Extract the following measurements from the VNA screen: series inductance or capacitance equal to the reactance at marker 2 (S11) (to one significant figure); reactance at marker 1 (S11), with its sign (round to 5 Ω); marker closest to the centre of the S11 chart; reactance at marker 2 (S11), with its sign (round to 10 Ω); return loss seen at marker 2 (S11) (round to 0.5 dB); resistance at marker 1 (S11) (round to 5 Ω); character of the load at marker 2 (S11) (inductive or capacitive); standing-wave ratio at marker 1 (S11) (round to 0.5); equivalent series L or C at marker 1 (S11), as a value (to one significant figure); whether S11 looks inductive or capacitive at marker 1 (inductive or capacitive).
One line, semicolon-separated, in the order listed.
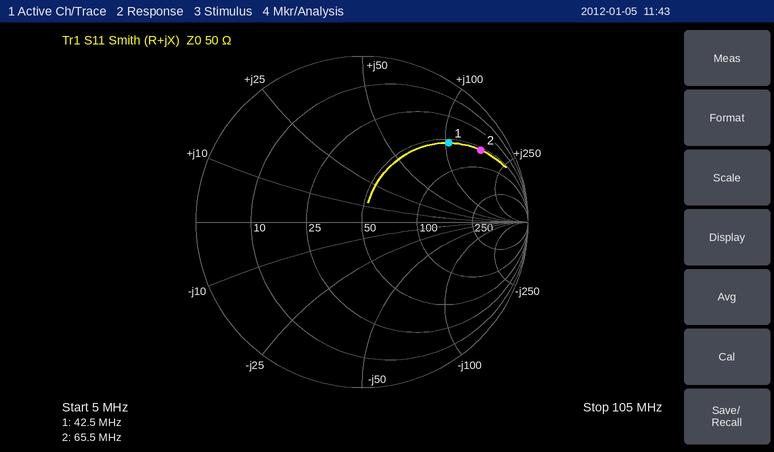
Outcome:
400 nH; +105 Ω; marker 1; +160 Ω; 1.5 dB; 55 Ω; inductive; 6.0; 400 nH; inductive
